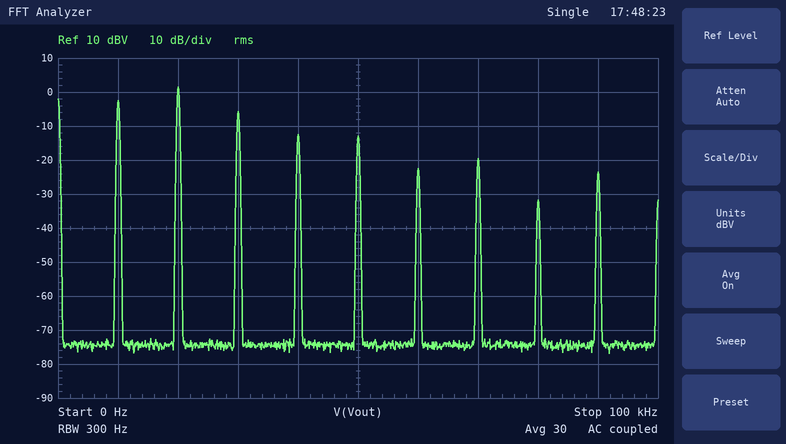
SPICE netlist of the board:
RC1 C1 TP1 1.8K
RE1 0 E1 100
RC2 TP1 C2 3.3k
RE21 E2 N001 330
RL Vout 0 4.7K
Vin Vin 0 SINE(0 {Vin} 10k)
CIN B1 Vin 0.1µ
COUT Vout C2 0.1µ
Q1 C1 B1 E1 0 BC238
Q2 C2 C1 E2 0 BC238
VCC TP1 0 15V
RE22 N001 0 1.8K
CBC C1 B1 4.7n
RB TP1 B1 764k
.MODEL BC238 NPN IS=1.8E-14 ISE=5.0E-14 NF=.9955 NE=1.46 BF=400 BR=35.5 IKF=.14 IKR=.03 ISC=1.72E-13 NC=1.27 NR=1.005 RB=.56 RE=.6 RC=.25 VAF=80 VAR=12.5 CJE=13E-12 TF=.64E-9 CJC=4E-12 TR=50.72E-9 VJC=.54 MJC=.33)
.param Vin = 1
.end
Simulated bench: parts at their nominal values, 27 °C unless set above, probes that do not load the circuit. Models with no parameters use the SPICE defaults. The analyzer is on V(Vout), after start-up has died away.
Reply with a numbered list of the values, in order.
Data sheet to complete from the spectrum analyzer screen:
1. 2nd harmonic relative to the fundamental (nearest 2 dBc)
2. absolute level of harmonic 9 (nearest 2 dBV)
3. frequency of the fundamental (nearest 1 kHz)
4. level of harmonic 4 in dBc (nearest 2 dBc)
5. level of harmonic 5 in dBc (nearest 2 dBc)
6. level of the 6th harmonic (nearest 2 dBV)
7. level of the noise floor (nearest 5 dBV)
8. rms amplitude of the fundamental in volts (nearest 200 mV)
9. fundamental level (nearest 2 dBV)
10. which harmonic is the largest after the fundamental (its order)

1. 4 dBc
2. -24 dBV
3. 10 kHz
4. -10 dBc
5. -10 dBc
6. -22 dBV
7. -75 dBV
8. 800 mV
9. -2 dBV
10. 2
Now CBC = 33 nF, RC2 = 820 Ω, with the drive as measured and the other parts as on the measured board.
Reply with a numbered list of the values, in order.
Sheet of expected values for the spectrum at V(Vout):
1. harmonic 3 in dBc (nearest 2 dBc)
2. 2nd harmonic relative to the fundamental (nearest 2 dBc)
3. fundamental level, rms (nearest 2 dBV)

1. -56 dBc
2. -42 dBc
3. -6 dBV
